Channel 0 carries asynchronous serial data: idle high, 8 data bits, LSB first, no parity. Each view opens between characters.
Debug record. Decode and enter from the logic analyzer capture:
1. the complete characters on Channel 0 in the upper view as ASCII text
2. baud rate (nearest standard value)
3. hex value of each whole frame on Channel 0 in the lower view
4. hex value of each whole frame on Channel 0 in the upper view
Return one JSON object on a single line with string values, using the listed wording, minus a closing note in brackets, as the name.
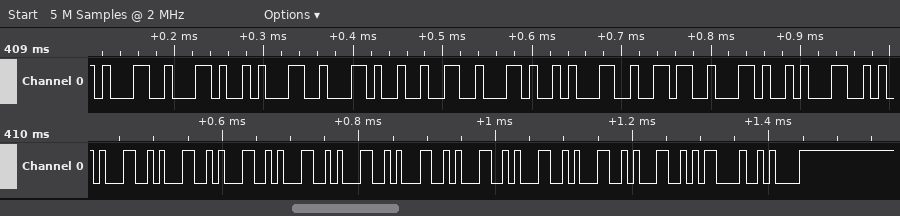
{"the complete characters on Channel 0 in the upper view as ASCII text": "\"1,1,2,16,1\"", "baud rate": "115200 baud", "hex value of each whole frame on Channel 0 in the lower view": "31, 31, 31, 31, 31, 31, 31, 31, 31, 31, 0D, 0A", "hex value of each whole frame on Channel 0 in the upper view": "31, 2C, 31, 2C, 32, 2C, 31, 36, 2C, 31"}
